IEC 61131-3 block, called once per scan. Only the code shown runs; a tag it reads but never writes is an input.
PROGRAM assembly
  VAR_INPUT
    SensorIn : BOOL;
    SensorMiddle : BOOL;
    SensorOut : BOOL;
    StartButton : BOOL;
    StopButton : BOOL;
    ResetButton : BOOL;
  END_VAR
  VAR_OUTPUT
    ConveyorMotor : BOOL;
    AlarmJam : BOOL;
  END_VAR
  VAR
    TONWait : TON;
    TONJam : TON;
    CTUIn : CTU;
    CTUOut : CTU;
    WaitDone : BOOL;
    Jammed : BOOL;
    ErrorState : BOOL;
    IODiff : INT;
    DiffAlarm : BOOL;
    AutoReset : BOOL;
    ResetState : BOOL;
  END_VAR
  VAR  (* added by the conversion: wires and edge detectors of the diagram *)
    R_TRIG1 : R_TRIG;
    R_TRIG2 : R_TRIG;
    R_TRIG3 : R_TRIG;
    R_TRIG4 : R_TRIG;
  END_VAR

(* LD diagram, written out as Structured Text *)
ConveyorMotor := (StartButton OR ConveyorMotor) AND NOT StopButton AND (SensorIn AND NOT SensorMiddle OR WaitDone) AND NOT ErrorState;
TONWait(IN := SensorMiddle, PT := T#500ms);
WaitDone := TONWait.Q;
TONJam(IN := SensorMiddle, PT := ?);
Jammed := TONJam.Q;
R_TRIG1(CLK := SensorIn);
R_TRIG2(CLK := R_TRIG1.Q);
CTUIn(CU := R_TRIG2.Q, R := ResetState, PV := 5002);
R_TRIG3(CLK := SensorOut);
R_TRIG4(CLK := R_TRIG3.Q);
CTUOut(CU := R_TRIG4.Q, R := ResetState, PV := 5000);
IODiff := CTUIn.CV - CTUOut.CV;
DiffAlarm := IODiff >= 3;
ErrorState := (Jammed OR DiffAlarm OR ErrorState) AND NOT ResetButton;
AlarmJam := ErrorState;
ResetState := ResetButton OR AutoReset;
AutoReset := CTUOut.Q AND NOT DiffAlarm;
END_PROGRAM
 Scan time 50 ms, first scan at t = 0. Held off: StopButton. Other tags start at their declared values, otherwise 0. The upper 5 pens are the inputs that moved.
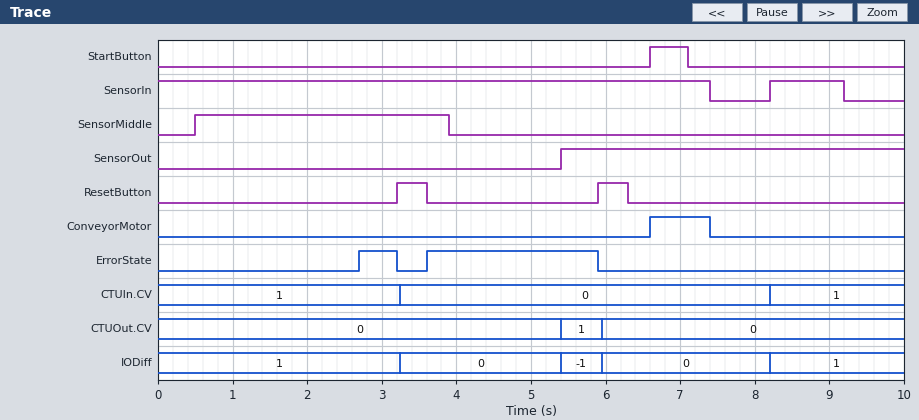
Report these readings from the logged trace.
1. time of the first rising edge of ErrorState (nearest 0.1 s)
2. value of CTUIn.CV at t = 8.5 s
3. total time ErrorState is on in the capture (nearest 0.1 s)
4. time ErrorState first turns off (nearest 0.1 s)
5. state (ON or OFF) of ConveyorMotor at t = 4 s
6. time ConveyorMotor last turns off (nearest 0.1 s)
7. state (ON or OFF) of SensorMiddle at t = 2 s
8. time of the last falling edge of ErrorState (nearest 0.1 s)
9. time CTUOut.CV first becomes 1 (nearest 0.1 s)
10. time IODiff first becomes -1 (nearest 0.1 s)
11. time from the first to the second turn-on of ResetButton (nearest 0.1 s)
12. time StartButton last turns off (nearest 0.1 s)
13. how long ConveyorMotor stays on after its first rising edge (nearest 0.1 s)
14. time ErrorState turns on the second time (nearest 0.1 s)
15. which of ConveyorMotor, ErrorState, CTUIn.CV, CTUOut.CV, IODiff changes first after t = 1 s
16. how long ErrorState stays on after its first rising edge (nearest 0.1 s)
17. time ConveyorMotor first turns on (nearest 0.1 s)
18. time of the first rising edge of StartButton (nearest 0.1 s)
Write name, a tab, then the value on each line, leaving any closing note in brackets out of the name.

time of the first rising edge of ErrorState	2.7 s
value of CTUIn.CV at t = 8.5 s	1
total time ErrorState is on in the capture	2.8 s
time ErrorState first turns off	3.2 s
state (ON or OFF) of ConveyorMotor at t = 4 s	OFF
time ConveyorMotor last turns off	7.4 s
state (ON or OFF) of SensorMiddle at t = 2 s	ON
time of the last falling edge of ErrorState	5.9 s
time CTUOut.CV first becomes 1	5.4 s
time IODiff first becomes -1	5.4 s
time from the first to the second turn-on of ResetButton	2.7 s
time StartButton last turns off	7.1 s
how long ConveyorMotor stays on after its first rising edge	0.8 s
time ErrorState turns on the second time	3.6 s
which of ConveyorMotor, ErrorState, CTUIn.CV, CTUOut.CV, IODiff changes first after t = 1 s	ErrorState
how long ErrorState stays on after its first rising edge	0.5 s
time ConveyorMotor first turns on	6.6 s
time of the first rising edge of StartButton	6.6 s
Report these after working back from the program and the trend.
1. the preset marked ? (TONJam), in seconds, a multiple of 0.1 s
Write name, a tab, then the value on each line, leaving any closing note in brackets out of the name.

the preset marked ? (TONJam), in seconds, a multiple of 0.1 s	2.2 s
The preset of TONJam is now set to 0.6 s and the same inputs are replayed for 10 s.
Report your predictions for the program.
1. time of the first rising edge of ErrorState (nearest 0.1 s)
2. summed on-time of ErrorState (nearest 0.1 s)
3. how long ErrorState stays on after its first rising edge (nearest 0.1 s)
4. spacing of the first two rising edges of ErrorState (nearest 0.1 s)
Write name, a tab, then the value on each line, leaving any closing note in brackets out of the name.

time of the first rising edge of ErrorState	1.1 s
summed on-time of ErrorState	4.4 s
how long ErrorState stays on after its first rising edge	2.1 s
spacing of the first two rising edges of ErrorState	2.5 s
